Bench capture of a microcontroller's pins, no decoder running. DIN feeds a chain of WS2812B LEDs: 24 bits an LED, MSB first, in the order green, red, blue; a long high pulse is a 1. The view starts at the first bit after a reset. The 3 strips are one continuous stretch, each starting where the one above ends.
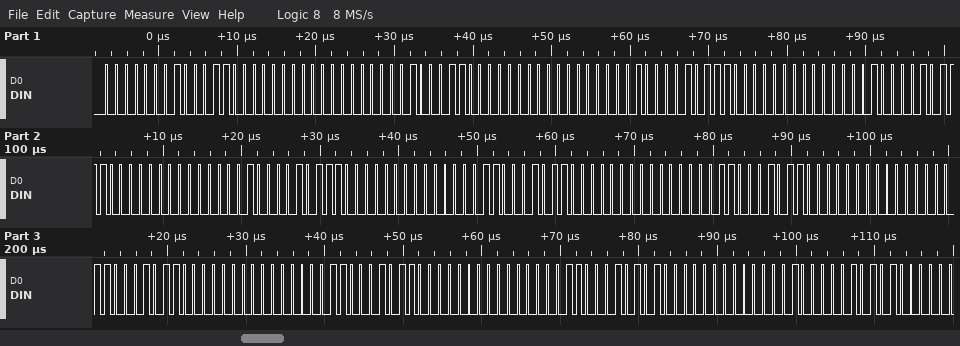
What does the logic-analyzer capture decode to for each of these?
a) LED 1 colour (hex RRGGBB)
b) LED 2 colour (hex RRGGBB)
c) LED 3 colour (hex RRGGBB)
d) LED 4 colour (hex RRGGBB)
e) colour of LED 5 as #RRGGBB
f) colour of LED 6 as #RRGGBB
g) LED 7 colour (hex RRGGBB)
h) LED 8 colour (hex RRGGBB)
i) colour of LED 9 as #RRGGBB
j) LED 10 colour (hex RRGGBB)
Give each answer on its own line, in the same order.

#180100
#180100
#170200
#170200
#170200
#160300
#160300
#160300
#160300
#150300
